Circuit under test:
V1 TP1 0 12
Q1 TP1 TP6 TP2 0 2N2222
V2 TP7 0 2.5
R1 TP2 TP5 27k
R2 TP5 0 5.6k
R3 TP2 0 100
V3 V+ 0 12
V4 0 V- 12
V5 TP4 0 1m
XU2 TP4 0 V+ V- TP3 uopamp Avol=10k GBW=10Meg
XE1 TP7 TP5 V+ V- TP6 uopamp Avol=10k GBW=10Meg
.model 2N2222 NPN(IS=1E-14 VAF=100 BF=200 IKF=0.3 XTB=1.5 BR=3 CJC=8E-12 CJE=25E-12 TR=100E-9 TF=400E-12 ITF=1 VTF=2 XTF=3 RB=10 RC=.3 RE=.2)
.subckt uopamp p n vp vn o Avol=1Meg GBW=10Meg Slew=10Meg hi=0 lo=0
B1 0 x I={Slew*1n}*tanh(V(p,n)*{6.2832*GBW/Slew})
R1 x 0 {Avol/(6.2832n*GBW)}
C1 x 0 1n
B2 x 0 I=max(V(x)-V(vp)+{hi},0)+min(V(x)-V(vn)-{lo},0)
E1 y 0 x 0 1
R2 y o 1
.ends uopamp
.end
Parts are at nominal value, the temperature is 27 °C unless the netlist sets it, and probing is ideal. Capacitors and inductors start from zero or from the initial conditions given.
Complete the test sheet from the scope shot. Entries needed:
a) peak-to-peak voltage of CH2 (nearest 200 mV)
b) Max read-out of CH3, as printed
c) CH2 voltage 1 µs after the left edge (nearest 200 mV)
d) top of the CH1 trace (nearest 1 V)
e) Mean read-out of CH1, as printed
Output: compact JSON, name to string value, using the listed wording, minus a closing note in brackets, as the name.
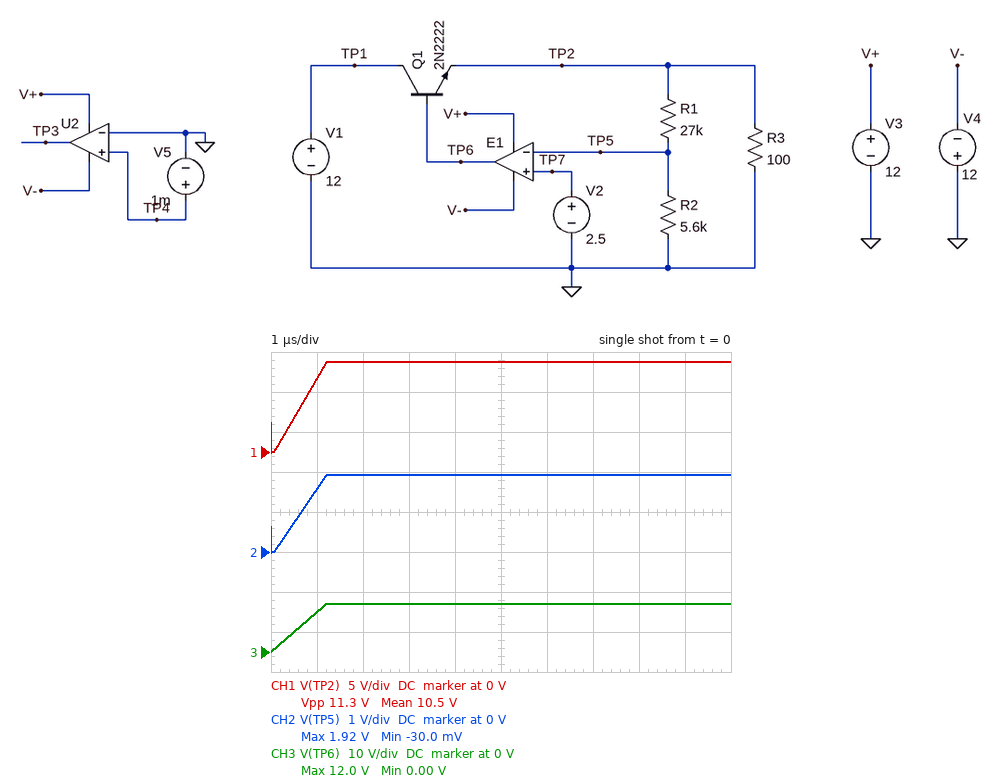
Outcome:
{"peak-to-peak voltage of CH2": "2.0 V", "Max read-out of CH3, as printed": "12.0 V", "CH2 voltage 1 µs after the left edge": "1.6 V", "top of the CH1 trace": "11 V", "Mean read-out of CH1, as printed": "10.5 V"}
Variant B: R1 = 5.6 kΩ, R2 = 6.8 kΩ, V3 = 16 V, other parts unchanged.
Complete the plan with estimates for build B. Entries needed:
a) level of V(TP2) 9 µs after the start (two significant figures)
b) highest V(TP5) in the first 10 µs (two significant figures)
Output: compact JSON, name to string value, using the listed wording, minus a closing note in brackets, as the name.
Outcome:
{"level of V(TP2) 9 µs after the start": "4.6 V", "highest V(TP5) in the first 10 µs": "2.5 V"}
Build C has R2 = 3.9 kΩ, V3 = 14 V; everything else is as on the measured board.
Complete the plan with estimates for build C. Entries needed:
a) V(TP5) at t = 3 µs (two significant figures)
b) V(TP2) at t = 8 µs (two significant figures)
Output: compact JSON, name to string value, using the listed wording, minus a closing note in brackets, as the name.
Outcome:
{"V(TP5) at t = 3 µs": "1.5 V", "V(TP2) at t = 8 µs": "12 V"}
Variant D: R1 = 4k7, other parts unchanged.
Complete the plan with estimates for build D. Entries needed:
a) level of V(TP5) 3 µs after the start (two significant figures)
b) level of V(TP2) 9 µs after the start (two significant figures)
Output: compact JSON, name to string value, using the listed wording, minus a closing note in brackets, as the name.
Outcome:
{"level of V(TP5) 3 µs after the start": "2.5 V", "level of V(TP2) 9 µs after the start": "4.6 V"}
